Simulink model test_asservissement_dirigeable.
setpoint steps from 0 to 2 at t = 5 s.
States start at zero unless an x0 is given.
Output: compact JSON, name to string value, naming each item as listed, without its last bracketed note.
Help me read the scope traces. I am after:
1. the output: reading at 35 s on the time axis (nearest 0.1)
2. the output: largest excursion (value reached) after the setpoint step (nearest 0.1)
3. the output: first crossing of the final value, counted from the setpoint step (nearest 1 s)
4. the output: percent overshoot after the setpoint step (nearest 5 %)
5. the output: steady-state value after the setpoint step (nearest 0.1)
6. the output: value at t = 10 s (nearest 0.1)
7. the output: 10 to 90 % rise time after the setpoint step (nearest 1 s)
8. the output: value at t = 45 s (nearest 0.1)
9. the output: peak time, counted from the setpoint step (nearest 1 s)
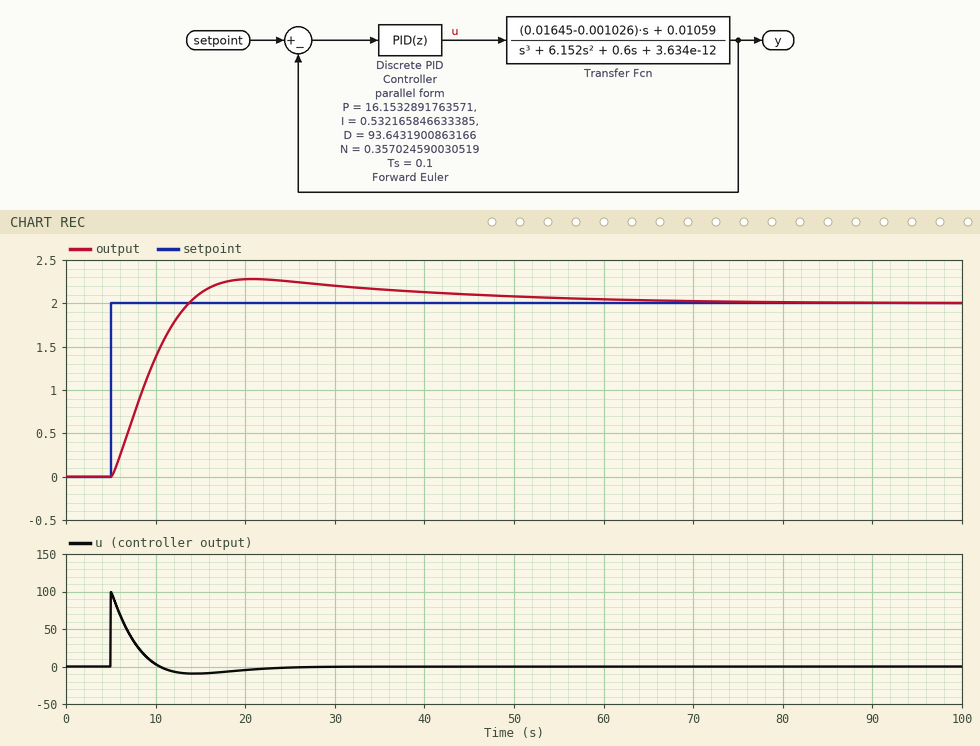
{"the output: reading at 35 s on the time axis": "2.2", "the output: largest excursion (value reached) after the setpoint step": "2.3", "the output: first crossing of the final value, counted from the setpoint step": "9 s", "the output: percent overshoot after the setpoint step": "15 %", "the output: steady-state value after the setpoint step": "2.0", "the output: value at t = 10 s": "1.4", "the output: 10 to 90 % rise time after the setpoint step": "6 s", "the output: value at t = 45 s": "2.1", "the output: peak time, counted from the setpoint step": "16 s"}
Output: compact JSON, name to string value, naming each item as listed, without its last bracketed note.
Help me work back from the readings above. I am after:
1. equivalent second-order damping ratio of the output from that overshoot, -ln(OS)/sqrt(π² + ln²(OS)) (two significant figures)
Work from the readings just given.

{"equivalent second-order damping ratio of the output from that overshoot, -ln(OS)/sqrt(π² + ln²(OS))": "0.52"}
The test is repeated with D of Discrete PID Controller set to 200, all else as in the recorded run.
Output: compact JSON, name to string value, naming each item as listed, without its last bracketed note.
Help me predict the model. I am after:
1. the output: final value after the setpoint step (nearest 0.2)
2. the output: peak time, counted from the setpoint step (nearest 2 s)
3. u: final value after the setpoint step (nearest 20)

{"the output: final value after the setpoint step": "2.0", "the output: peak time, counted from the setpoint step": "36 s", "u: final value after the setpoint step": "0"}
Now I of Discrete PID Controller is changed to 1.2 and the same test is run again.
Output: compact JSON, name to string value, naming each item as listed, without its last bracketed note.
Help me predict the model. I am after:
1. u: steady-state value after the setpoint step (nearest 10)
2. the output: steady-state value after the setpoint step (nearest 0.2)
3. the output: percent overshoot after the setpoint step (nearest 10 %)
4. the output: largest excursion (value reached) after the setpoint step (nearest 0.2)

{"u: steady-state value after the setpoint step": "0", "the output: steady-state value after the setpoint step": "2.0", "the output: percent overshoot after the setpoint step": "20 %", "the output: largest excursion (value reached) after the setpoint step": "2.4"}
